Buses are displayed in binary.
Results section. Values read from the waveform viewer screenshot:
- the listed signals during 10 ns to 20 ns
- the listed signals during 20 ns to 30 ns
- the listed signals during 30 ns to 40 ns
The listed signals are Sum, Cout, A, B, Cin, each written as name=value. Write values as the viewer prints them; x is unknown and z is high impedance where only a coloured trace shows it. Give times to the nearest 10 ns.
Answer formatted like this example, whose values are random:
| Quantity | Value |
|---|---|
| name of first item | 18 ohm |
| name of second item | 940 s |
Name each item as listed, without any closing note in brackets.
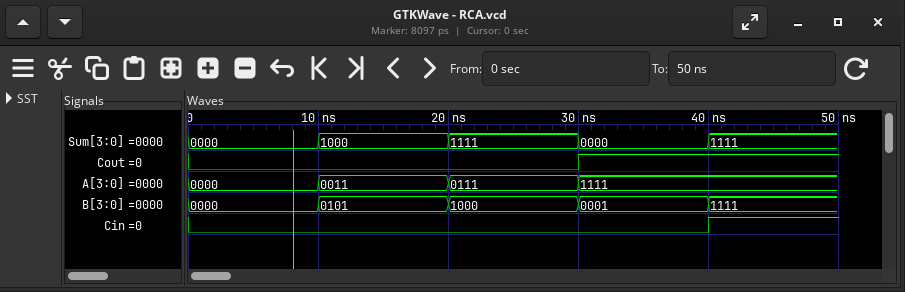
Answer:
| Quantity | Value |
|---|---|
| the listed signals during 10 ns to 20 ns | Sum=1000, Cout=0, A=0011, B=0101, Cin=0 |
| the listed signals during 20 ns to 30 ns | Sum=1111, Cout=0, A=0111, B=1000, Cin=0 |
| the listed signals during 30 ns to 40 ns | Sum=0000, Cout=1, A=1111, B=0001, Cin=0 |
